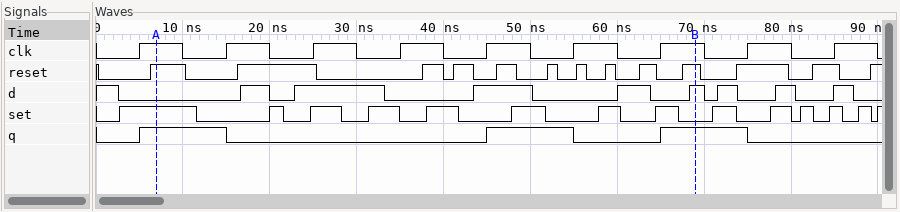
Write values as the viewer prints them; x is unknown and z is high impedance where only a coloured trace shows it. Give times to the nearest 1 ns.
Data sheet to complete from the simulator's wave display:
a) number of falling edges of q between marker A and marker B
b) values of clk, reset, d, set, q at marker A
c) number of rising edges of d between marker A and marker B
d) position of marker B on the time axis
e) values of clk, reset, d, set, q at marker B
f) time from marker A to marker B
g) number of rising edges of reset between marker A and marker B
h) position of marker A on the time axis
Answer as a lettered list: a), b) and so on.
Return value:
a) 2
b) clk=1, reset=1, d=0, set=1, q=1
c) 5
d) 69 ns
e) clk=1, reset=1, d=1, set=0, q=1
f) 62 ns
g) 9
h) 7 ns
